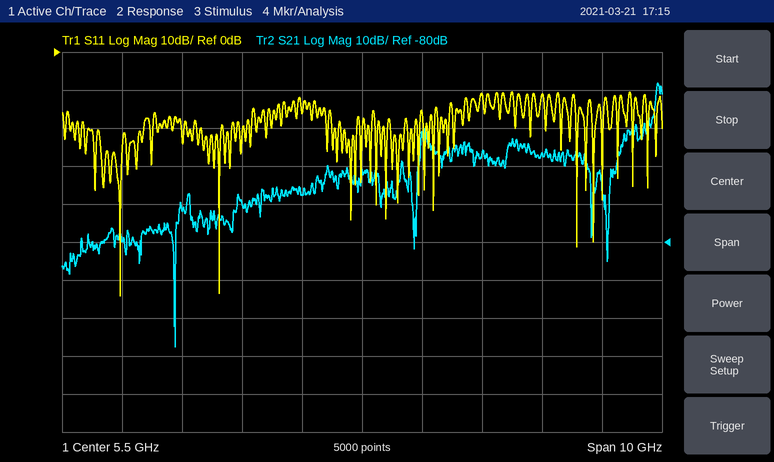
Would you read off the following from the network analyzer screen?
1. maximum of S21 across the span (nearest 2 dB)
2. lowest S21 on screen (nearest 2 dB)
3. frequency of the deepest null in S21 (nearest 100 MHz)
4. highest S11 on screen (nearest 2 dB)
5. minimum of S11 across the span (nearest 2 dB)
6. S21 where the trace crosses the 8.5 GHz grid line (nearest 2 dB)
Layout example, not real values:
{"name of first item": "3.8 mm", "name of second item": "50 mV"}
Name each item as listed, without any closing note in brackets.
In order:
{"maximum of S21 across the span": "-38 dB", "lowest S21 on screen": "-108 dB", "frequency of the deepest null in S21": "2.4 GHz", "highest S11 on screen": "-10 dB", "minimum of S11 across the span": "-64 dB", "S21 where the trace crosses the 8.5 GHz grid line": "-56 dB"}
